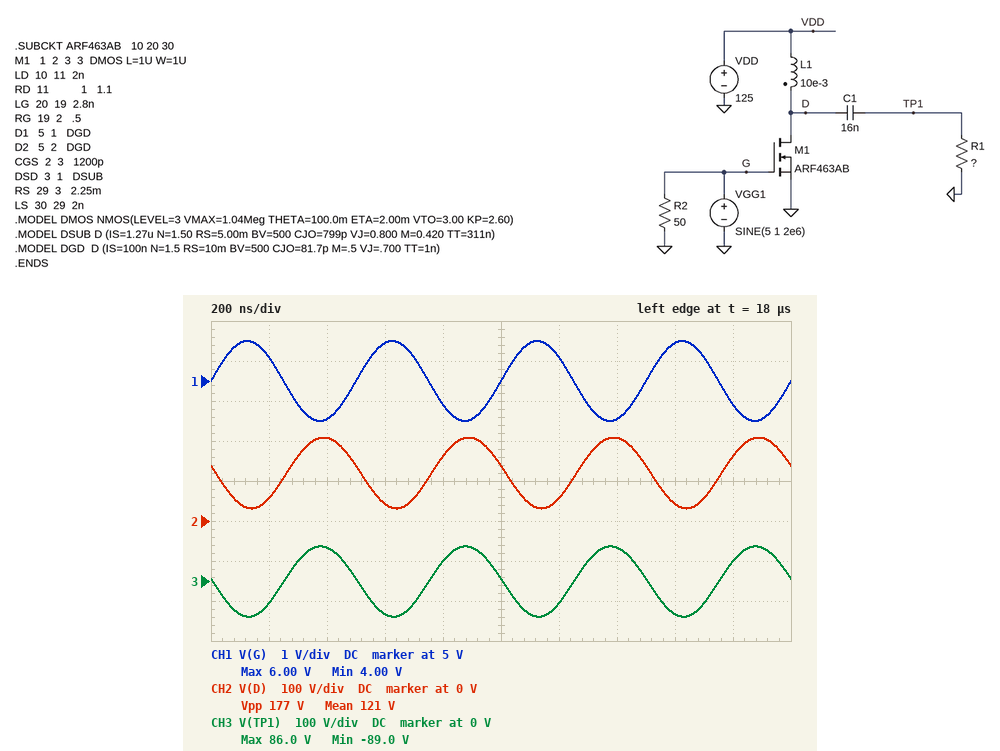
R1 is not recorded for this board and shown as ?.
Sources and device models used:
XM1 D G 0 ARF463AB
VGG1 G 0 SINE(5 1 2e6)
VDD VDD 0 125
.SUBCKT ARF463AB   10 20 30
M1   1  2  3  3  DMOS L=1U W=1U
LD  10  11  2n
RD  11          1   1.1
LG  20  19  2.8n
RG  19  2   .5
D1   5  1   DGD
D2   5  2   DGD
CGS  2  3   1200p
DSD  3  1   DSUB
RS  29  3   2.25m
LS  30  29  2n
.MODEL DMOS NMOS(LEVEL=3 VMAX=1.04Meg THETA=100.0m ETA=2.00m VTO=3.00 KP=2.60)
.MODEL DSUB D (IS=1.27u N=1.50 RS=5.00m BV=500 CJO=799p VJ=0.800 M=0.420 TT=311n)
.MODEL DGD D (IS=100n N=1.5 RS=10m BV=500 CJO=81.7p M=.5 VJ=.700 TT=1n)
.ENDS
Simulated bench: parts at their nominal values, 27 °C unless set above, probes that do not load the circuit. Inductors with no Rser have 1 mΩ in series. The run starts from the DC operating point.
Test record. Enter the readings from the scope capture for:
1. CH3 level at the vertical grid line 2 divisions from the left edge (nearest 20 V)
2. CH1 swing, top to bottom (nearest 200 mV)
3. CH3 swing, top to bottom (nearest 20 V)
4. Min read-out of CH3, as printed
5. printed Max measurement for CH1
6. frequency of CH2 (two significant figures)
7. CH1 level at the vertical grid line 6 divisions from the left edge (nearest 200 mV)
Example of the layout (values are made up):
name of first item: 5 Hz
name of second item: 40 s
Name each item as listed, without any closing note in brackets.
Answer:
CH3 level at the vertical grid line 2 divisions from the left edge: 80 V
CH1 swing, top to bottom: 2.0 V
CH3 swing, top to bottom: 180 V
Min read-out of CH3, as printed: -89.0 V
printed Max measurement for CH1: 6.00 V
frequency of CH2: 2.0 MHz
CH1 level at the vertical grid line 6 divisions from the left edge: 5.6 V
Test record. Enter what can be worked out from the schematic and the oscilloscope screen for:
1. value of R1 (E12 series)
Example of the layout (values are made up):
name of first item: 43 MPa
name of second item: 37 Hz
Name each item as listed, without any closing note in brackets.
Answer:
value of R1: 39 Ω
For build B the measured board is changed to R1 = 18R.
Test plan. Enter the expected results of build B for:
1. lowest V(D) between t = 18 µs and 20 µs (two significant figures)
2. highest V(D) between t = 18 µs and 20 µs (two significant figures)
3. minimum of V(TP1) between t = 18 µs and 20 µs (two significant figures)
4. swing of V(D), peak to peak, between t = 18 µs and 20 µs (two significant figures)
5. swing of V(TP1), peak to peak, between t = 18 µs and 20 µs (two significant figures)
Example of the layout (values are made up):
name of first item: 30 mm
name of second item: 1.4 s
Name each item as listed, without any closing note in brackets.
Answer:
lowest V(D) between t = 18 µs and 20 µs: 63 V
highest V(D) between t = 18 µs and 20 µs: 170 V
minimum of V(TP1) between t = 18 µs and 20 µs: -54 V
swing of V(D), peak to peak, between t = 18 µs and 20 µs: 110 V
swing of V(TP1), peak to peak, between t = 18 µs and 20 µs: 100 V
